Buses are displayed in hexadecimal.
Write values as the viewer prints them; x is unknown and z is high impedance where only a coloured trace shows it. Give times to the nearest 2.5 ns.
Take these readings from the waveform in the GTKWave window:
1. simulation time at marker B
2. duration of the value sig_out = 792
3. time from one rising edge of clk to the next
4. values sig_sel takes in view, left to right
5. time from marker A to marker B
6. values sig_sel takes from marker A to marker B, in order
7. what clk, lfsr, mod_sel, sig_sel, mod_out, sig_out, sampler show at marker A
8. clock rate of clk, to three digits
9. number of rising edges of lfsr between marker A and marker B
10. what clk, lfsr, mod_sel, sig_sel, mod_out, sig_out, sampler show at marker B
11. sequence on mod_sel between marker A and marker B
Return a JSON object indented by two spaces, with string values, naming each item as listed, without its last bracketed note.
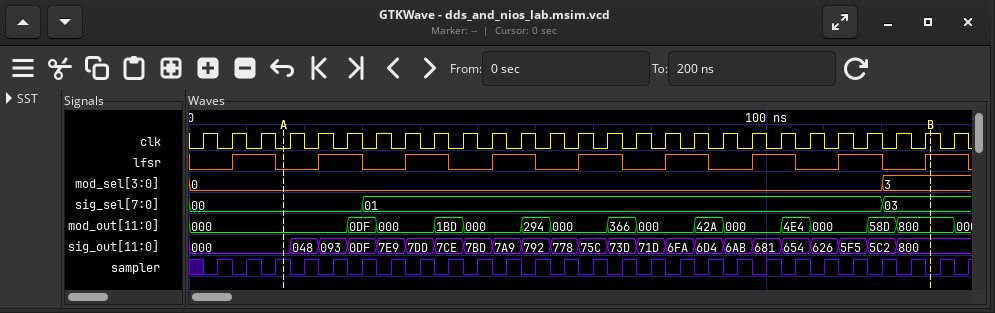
{
  "simulation time at marker B": "127.5 ns",
  "duration of the value sig_out = 792": "5 ns",
  "time from one rising edge of clk to the next": "5 ns",
  "values sig_sel takes in view, left to right": "00, 01, 03",
  "time from marker A to marker B": "112.5 ns",
  "values sig_sel takes from marker A to marker B, in order": "00, 01, 03",
  "what clk, lfsr, mod_sel, sig_sel, mod_out, sig_out, sampler show at marker A": "clk=0, lfsr=0, mod_sel=0, sig_sel=00, mod_out=000, sig_out=000, sampler=1",
  "clock rate of clk, to three digits": "200 MHz",
  "number of rising edges of lfsr between marker A and marker B": "8",
  "what clk, lfsr, mod_sel, sig_sel, mod_out, sig_out, sampler show at marker B": "clk=1, lfsr=1, mod_sel=3, sig_sel=03, mod_out=800, sig_out=800, sampler=0",
  "sequence on mod_sel between marker A and marker B": "0, 3"
}
